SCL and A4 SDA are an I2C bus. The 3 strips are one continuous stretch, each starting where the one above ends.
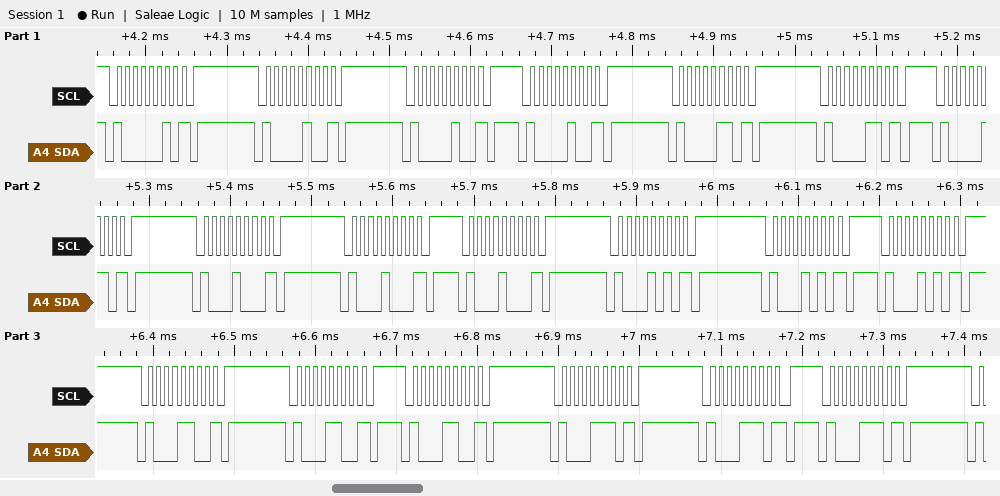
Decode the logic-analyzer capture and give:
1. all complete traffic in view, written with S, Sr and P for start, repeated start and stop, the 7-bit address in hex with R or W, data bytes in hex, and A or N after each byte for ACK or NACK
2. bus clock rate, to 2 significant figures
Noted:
S 41W N P S 42W N P S 42W N P S 42W N P S 43W N P S 43W N P S 43W N P S 44W N P S 44W N P S 44W N P S 45W N P S 45W N P S 45W N P S 46W N P S 46W N P S 46W N P S 47W N P S 47W N P S 47W N P
100 kHz
